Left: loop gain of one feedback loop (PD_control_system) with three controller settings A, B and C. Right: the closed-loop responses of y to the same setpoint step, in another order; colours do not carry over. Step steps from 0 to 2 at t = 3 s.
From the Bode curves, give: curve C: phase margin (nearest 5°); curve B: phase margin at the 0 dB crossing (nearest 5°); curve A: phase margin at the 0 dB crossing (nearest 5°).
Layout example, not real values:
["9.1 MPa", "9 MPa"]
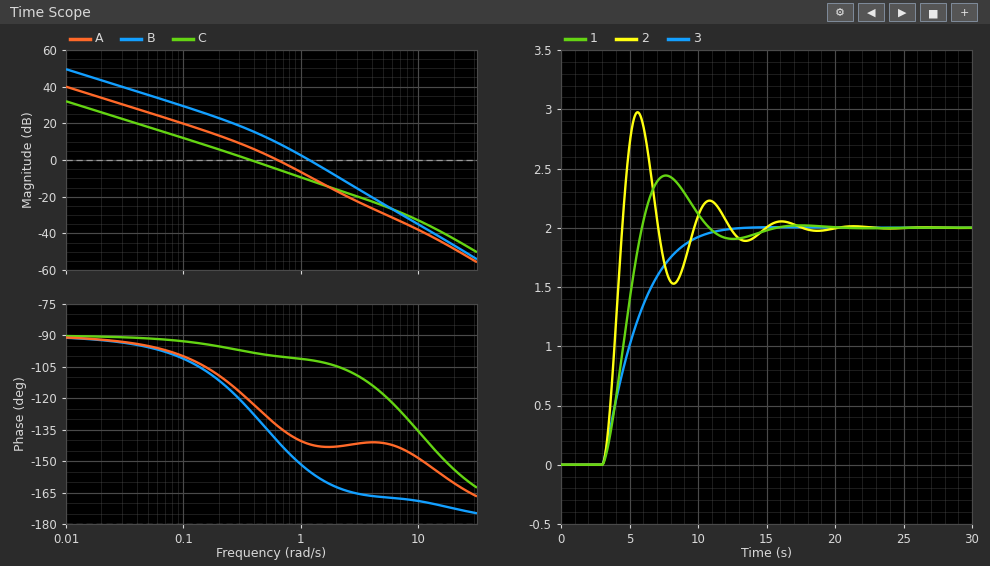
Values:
["80°", "25°", "45°"]
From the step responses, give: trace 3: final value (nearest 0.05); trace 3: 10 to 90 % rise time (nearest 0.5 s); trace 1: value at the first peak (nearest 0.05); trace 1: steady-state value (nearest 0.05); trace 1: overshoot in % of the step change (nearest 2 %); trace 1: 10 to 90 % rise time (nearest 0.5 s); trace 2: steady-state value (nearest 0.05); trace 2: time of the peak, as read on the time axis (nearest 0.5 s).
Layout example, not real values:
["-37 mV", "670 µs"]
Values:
["2.00", "5.0 s", "2.45", "2.00", "22 %", "2.0 s", "2.00", "5.5 s"]
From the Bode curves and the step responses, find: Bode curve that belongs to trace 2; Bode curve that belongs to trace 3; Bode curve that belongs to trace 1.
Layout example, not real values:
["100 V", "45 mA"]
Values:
["B", "C", "A"]
